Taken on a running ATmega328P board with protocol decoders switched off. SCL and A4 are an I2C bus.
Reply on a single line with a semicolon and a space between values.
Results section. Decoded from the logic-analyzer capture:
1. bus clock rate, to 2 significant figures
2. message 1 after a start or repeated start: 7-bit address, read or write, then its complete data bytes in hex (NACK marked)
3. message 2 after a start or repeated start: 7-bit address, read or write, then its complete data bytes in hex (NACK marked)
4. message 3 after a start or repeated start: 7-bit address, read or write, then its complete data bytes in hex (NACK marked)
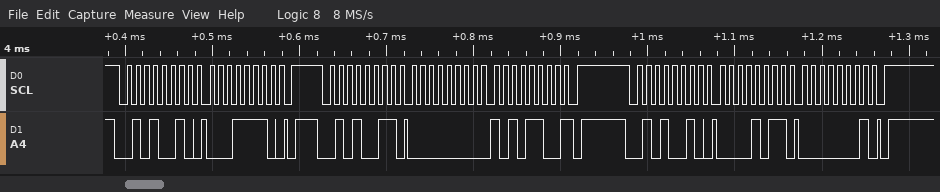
100 kHz; 0x29 write: 1E; 0x29 read: 00 AC NACK; 0x29 write: 0B 01
